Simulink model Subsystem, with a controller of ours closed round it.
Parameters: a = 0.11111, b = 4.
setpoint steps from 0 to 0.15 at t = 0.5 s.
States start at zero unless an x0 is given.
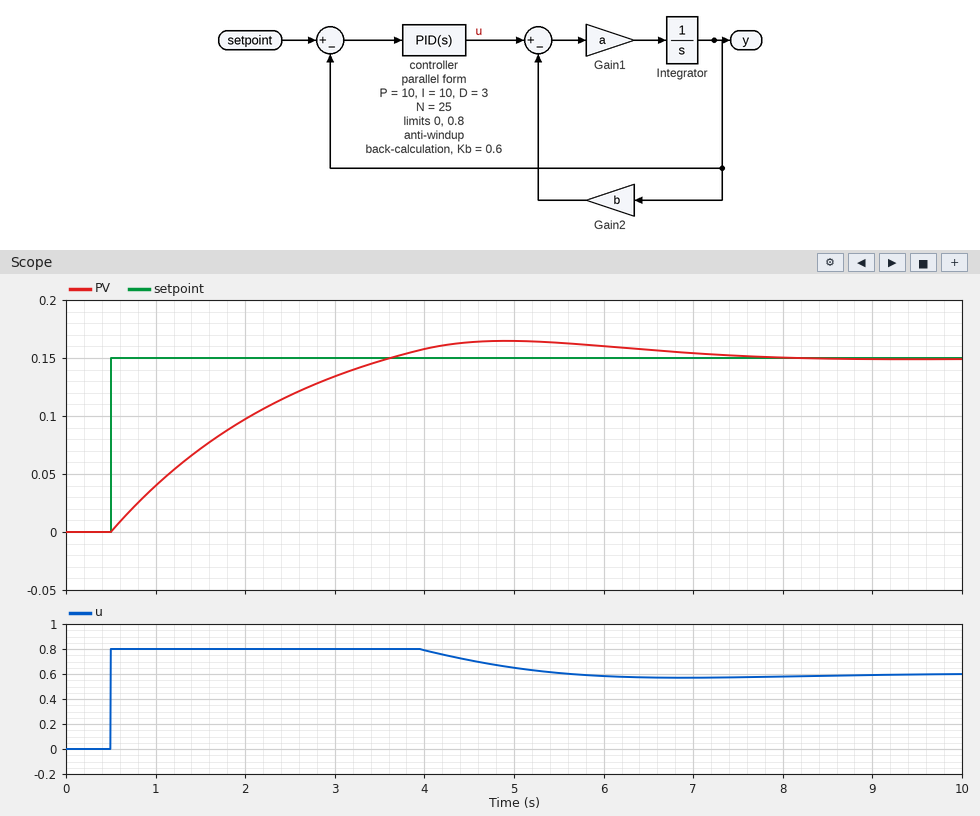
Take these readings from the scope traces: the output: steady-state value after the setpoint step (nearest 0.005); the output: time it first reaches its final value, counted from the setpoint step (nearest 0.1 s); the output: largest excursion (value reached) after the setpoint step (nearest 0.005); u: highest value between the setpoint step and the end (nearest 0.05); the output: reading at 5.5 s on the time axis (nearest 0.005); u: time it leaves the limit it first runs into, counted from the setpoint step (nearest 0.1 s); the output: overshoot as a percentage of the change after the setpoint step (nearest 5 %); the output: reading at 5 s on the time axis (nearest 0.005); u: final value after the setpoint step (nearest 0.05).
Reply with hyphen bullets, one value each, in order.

- 0.150
- 3.1 s
- 0.165
- 0.80
- 0.165
- 3.5 s
- 10 %
- 0.165
- 0.60
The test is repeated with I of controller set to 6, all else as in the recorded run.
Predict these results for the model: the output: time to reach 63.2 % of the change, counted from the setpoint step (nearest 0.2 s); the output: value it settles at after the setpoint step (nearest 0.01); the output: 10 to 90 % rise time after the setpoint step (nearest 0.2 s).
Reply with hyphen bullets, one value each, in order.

- 1.4 s
- 0.15
- 2.4 s
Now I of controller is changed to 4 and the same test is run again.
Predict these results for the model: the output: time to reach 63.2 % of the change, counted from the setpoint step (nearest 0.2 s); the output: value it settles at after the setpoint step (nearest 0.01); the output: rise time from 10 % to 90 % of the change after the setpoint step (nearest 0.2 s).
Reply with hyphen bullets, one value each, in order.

- 1.6 s
- 0.15
- 3.2 s
